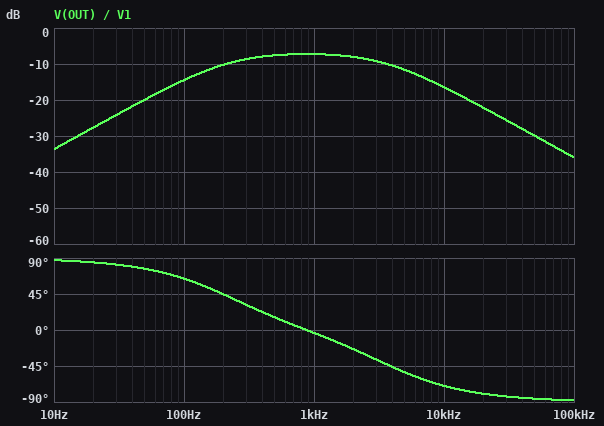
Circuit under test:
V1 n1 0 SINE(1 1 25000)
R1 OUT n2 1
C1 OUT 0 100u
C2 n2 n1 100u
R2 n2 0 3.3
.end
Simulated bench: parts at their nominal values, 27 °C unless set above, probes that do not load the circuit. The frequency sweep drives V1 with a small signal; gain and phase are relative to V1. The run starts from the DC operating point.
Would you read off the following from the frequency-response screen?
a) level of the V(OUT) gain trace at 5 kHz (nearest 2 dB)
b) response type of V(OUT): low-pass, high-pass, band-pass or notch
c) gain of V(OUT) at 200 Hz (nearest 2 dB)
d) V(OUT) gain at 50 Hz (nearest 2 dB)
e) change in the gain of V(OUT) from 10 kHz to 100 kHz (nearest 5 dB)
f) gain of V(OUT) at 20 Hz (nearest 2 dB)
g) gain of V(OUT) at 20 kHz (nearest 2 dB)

-12 dB
band-pass
-10 dB
-20 dB
-20 dB
-28 dB
-22 dB
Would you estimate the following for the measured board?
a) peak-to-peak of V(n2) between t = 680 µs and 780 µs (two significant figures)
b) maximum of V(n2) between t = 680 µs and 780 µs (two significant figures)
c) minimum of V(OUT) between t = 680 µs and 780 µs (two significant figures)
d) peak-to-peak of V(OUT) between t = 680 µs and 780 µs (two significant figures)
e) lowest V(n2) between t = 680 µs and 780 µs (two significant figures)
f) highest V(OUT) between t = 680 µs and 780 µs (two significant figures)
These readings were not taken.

2.0 V
990 mV
-65 mV
130 mV
-990 mV
62 mV
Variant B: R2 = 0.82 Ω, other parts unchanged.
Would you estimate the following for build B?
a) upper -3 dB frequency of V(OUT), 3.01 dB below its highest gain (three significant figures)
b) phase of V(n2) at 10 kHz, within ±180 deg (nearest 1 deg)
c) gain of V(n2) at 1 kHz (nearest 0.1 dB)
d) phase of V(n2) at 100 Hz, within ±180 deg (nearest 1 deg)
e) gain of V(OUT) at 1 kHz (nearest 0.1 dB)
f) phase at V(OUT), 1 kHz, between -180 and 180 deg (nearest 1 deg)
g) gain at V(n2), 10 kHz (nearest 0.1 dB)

5.67 kHz
19 deg
-9.4 dB
84 deg
-10.8 dB
22 deg
-0.7 dB
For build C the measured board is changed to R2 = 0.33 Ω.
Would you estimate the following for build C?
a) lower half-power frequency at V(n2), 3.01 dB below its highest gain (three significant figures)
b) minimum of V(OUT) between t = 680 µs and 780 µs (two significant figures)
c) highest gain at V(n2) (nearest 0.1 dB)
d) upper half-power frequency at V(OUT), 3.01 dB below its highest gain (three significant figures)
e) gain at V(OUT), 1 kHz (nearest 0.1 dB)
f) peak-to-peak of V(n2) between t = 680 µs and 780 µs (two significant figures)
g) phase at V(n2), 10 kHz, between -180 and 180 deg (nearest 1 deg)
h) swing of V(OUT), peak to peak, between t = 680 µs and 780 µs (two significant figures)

6.71 kHz
-61 mV
0 dB
8.87 kHz
-16.3 dB
1.9 V
32 deg
120 mV
